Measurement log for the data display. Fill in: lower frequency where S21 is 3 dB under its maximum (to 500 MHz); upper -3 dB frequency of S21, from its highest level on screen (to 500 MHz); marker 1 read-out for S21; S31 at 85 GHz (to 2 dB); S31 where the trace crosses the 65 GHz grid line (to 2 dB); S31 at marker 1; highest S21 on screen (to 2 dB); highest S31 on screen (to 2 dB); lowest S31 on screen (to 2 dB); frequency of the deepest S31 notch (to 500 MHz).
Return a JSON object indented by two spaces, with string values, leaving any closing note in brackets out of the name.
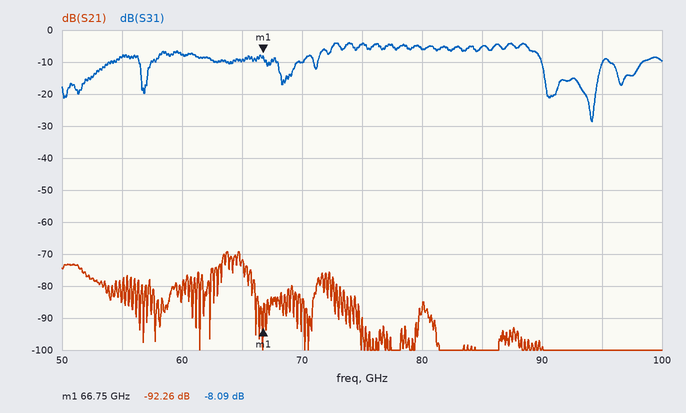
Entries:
{
  "lower frequency where S21 is 3 dB under its maximum": "63.5 GHz",
  "upper -3 dB frequency of S21, from its highest level on screen": "64.0 GHz",
  "marker 1 read-out for S21": "-92.26 dB",
  "S31 at 85 GHz": "-6 dB",
  "S31 where the trace crosses the 65 GHz grid line": "-10 dB",
  "S31 at marker 1": "-8.09 dB",
  "highest S21 on screen": "-70 dB",
  "highest S31 on screen": "-4 dB",
  "lowest S31 on screen": "-28 dB",
  "frequency of the deepest S31 notch": "94.0 GHz"
}
